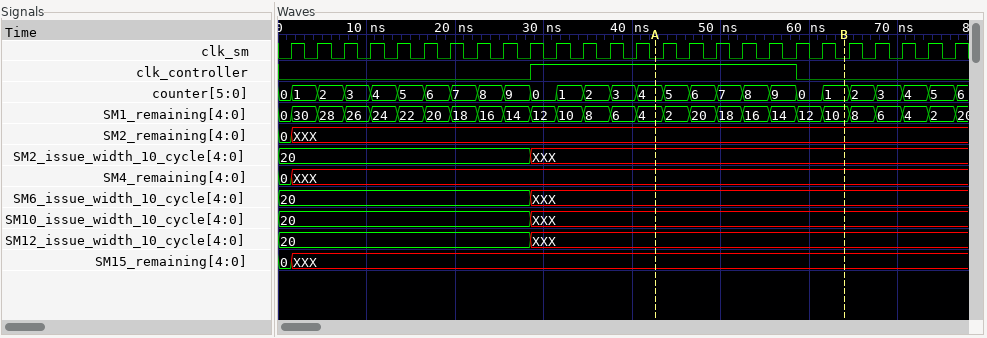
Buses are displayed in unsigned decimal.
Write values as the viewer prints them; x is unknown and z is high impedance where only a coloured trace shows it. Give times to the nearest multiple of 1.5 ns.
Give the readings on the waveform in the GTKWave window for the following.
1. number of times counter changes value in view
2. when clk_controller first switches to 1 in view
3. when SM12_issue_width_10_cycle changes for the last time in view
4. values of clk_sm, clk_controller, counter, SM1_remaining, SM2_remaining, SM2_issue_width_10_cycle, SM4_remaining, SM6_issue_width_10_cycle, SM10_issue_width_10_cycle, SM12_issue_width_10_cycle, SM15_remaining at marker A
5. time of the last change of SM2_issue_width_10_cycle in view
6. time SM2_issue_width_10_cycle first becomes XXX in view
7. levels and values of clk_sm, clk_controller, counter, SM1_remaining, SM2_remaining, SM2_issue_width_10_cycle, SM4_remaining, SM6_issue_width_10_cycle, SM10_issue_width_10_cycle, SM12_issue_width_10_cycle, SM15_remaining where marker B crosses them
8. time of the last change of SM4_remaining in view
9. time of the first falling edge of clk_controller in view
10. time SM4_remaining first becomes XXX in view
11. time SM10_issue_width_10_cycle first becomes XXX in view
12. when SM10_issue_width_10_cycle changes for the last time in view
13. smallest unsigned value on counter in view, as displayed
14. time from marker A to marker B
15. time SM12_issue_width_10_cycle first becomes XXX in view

26
28.5 ns
28.5 ns
clk_sm=0, clk_controller=1, counter=4, SM1_remaining=4, SM2_remaining=XXX, SM2_issue_width_10_cycle=XXX, SM4_remaining=XXX, SM6_issue_width_10_cycle=XXX, SM10_issue_width_10_cycle=XXX, SM12_issue_width_10_cycle=XXX, SM15_remaining=XXX
28.5 ns
28.5 ns
clk_sm=0, clk_controller=0, counter=1, SM1_remaining=10, SM2_remaining=XXX, SM2_issue_width_10_cycle=XXX, SM4_remaining=XXX, SM6_issue_width_10_cycle=XXX, SM10_issue_width_10_cycle=XXX, SM12_issue_width_10_cycle=XXX, SM15_remaining=XXX
1.5 ns
58.5 ns
1.5 ns
28.5 ns
28.5 ns
0
21 ns
28.5 ns
